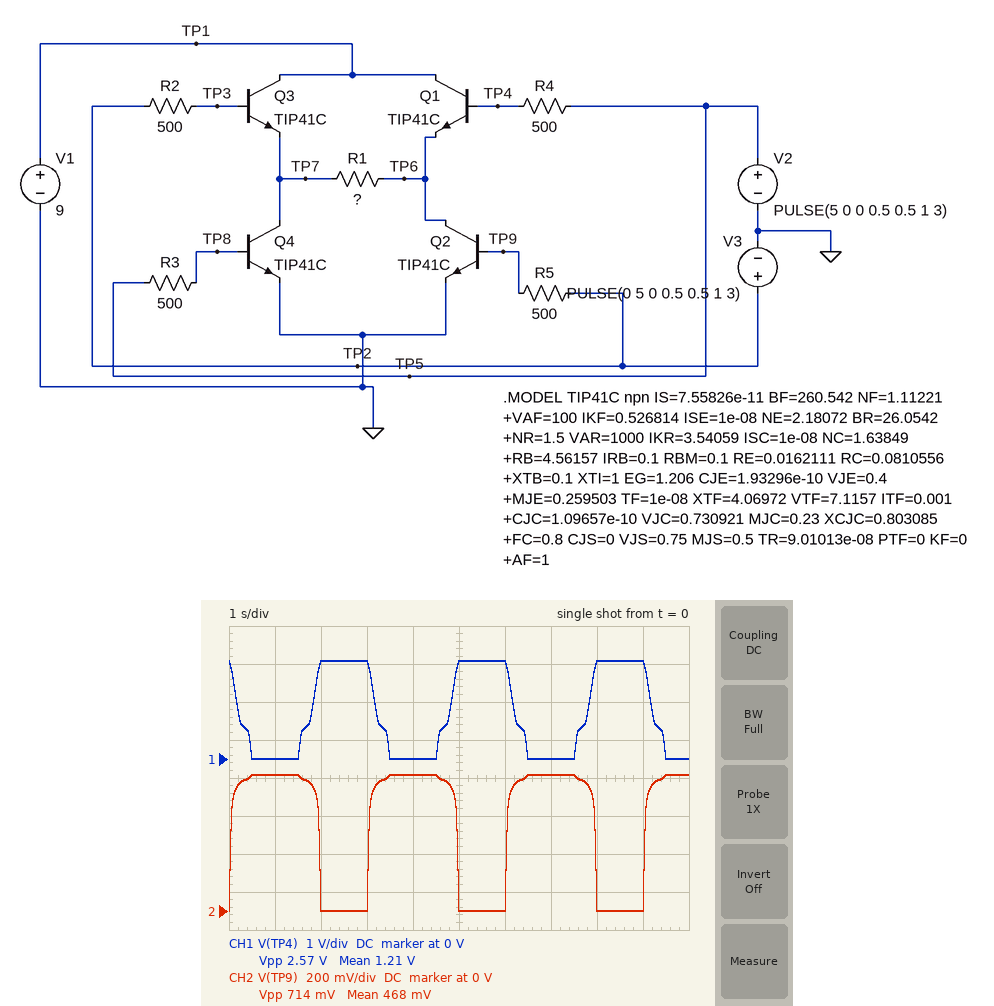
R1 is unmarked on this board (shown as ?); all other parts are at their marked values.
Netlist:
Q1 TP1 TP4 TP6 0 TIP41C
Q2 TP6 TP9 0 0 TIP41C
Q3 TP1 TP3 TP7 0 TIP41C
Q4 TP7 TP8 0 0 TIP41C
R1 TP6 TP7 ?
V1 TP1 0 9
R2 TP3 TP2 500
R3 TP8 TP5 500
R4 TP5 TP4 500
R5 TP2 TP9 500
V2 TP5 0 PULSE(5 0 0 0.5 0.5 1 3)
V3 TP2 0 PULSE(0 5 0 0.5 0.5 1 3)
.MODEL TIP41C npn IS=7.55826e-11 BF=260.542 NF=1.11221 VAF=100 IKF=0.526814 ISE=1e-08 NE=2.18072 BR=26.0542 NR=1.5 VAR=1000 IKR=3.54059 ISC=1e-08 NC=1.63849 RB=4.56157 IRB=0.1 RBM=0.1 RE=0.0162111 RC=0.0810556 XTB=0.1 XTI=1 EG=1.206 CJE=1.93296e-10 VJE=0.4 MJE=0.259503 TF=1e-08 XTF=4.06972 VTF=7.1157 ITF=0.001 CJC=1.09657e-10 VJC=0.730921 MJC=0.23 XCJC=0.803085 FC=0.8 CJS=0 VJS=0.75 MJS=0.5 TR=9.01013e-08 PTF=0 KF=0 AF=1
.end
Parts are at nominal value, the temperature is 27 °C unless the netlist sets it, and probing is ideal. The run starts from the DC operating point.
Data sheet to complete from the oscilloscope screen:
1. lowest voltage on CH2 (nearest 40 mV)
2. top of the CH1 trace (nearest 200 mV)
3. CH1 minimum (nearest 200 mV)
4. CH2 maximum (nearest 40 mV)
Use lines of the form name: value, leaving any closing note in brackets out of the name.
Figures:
lowest voltage on CH2: 0 V
top of the CH1 trace: 2.6 V
CH1 minimum: 0 V
CH2 maximum: 720 mV
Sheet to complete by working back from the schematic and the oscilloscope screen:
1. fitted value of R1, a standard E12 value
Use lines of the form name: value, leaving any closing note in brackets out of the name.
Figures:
fitted value of R1, a standard E12 value: 3.3 Ω
